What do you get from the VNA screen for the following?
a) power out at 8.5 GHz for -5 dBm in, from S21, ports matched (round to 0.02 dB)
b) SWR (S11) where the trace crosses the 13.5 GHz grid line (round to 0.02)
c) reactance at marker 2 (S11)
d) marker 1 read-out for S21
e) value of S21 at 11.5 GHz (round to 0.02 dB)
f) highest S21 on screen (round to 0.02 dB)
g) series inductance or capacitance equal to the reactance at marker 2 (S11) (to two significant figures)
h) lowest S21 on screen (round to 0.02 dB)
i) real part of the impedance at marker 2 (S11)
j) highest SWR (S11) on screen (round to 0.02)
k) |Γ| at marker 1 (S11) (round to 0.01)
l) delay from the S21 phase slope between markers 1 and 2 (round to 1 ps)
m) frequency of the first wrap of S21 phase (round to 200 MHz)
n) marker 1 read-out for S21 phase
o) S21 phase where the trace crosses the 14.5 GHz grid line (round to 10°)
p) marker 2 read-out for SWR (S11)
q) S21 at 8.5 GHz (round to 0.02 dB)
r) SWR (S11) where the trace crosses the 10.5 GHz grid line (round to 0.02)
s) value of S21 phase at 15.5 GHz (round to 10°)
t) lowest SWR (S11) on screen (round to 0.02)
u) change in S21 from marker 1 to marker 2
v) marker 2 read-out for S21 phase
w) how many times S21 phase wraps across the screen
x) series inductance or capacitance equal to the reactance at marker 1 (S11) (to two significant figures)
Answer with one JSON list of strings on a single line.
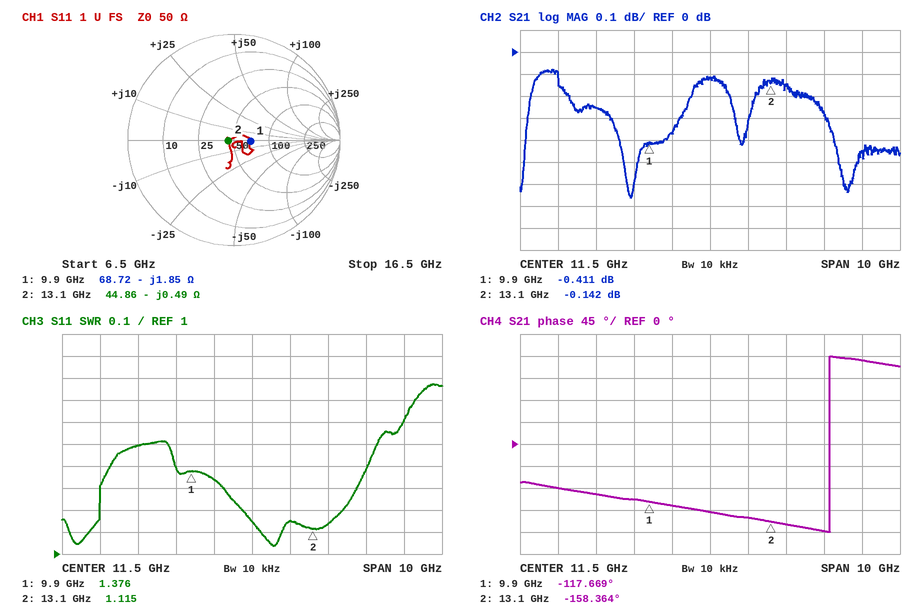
["-5.26 dBm", "1.14", "-0.49 Ω", "-0.411 dB", "-0.12 dB", "-0.08 dB", "25 pF", "-0.66 dB", "44.86 Ω", "1.78", "0.16", "35 ps", "14.6 GHz", "-117.669°", "-180°", "1.115", "-0.26 dB", "1.34", "170°", "1.04", "0.269 dB", "-158.364°", "1", "8.7 pF"]
